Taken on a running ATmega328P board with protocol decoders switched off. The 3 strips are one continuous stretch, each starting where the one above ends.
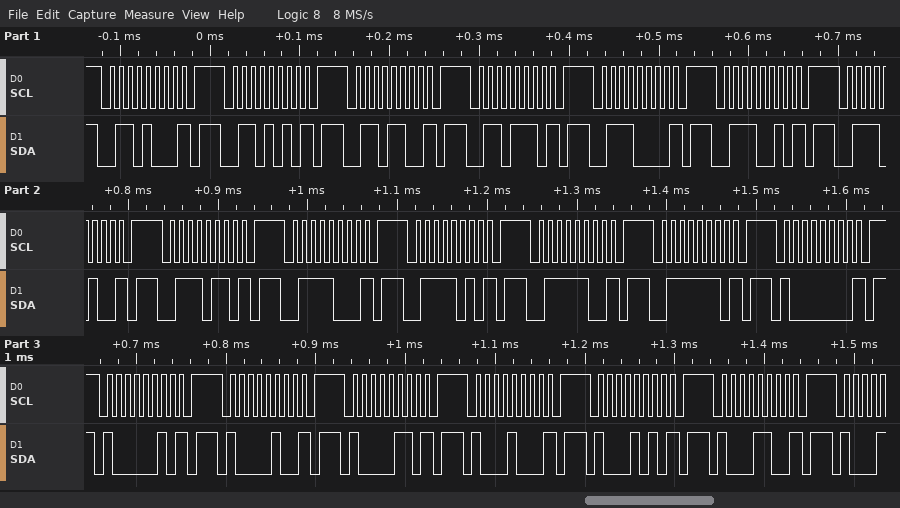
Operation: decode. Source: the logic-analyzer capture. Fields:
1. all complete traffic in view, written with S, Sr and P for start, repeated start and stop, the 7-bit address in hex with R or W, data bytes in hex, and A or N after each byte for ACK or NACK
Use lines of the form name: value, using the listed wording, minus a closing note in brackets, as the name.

all complete traffic in view, written with S, Sr and P for start, repeated start and stop, the 7-bit address in hex with R or W, data bytes in hex, and A or N after each byte for ACK or NACK: S 34W N P S 35W N P S 36W N P S 37W N P S 38W N P S 39W N P S 3AW N P S 3BW N P S 3CW N P S 3DW N P S 3EW N P S 3FW N P S 40W N P S 41W N P S 42W N P S 43W N P S 44W N P S 45W N P S 46W N P
